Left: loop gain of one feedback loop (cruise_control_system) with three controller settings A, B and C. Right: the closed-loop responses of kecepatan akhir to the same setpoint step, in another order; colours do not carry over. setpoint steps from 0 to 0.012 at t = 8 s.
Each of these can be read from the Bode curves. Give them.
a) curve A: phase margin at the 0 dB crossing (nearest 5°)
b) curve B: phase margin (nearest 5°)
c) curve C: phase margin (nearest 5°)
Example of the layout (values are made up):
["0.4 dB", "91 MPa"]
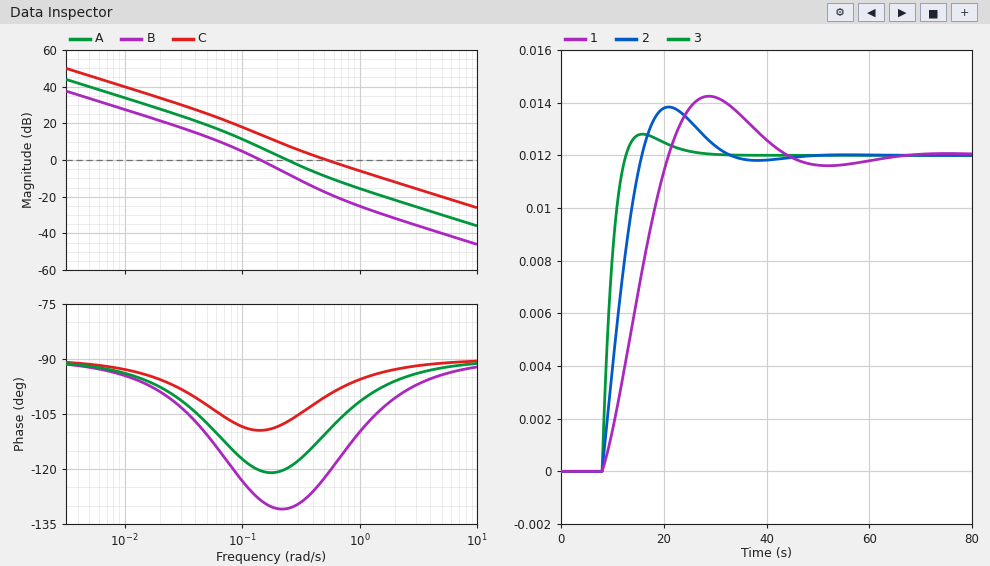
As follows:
["60°", "50°", "80°"]
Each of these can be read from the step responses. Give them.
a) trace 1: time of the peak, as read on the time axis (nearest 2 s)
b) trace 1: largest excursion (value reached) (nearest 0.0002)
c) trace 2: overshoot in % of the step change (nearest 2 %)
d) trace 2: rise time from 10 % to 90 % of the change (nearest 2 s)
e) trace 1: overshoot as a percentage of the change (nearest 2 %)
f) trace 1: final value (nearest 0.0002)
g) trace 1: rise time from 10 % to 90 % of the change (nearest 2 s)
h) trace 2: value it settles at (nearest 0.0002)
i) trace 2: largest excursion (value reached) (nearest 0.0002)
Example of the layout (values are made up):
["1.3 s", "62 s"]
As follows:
["28 s", "0.0142", "16 %", "6 s", "18 %", "0.0120", "10 s", "0.0120", "0.0138"]
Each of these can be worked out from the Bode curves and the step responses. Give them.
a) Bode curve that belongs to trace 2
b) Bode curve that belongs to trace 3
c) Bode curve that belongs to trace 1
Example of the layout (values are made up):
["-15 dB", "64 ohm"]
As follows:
["A", "C", "B"]
